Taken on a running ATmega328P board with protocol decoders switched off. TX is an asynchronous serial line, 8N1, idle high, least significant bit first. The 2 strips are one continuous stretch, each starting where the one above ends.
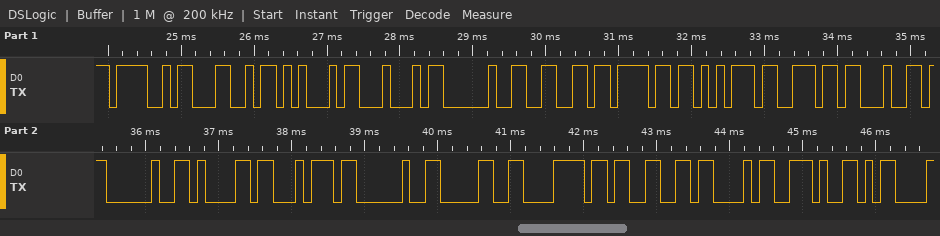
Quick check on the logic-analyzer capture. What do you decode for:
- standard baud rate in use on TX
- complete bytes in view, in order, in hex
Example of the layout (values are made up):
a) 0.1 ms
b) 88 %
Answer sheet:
a) 9600 baud
b) 0x4F 0x4C 0x45 0x44 0x20 0x66 0x6F 0x75 0x6E 0x64 0x20 0x61 0x74 0x20 0x30 0x78 0x33 0x43 0x2E 0x0D
